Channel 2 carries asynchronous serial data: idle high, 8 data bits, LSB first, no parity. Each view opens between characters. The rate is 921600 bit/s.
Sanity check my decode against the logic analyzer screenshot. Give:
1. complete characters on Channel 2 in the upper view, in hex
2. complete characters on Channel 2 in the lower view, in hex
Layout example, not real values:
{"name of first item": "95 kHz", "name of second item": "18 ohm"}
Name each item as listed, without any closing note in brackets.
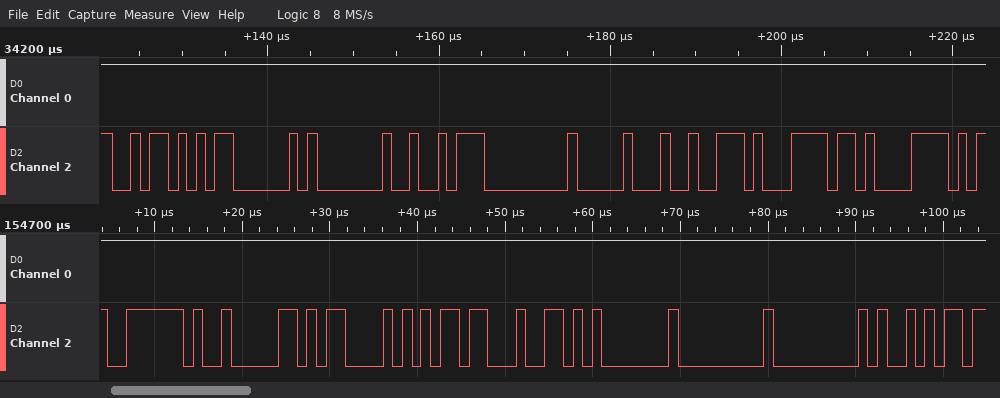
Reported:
{"complete characters on Channel 2 in the upper view, in hex": "5A, 03, 01, D2, 00, 10, 72, BC, E1", "complete characters on Channel 2 in the lower view, in hex": "7E, 82, 0D, B5, 64, 01, 00, 00, A9"}
